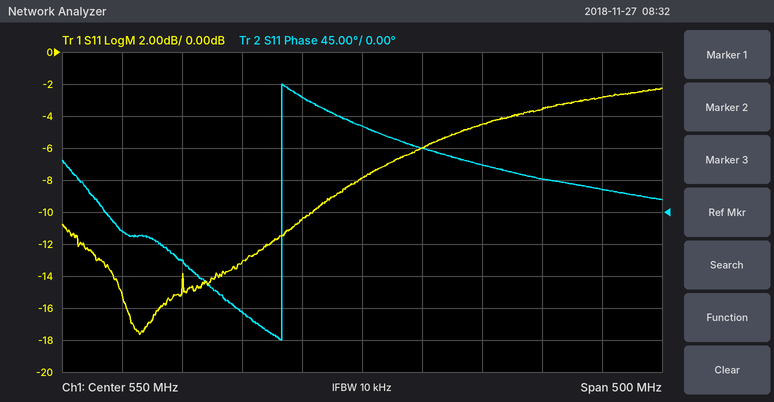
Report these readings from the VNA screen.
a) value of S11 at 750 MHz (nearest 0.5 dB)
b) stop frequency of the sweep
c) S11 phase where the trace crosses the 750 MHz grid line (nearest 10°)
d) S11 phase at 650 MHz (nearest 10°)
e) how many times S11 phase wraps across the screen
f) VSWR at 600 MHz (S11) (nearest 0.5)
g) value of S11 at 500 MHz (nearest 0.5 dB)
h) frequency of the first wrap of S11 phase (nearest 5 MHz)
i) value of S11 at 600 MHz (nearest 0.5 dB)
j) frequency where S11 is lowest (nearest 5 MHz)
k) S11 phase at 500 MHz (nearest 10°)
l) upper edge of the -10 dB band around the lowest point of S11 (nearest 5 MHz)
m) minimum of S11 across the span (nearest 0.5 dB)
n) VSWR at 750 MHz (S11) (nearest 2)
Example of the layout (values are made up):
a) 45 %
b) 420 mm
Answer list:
a) -3.0 dB
b) 800 MHz
c) 30°
d) 70°
e) 1
f) 3.0
g) -10.5 dB
h) 485 MHz
i) -6.0 dB
j) 365 MHz
k) 160°
l) 510 MHz
m) -17.5 dB
n) 6
